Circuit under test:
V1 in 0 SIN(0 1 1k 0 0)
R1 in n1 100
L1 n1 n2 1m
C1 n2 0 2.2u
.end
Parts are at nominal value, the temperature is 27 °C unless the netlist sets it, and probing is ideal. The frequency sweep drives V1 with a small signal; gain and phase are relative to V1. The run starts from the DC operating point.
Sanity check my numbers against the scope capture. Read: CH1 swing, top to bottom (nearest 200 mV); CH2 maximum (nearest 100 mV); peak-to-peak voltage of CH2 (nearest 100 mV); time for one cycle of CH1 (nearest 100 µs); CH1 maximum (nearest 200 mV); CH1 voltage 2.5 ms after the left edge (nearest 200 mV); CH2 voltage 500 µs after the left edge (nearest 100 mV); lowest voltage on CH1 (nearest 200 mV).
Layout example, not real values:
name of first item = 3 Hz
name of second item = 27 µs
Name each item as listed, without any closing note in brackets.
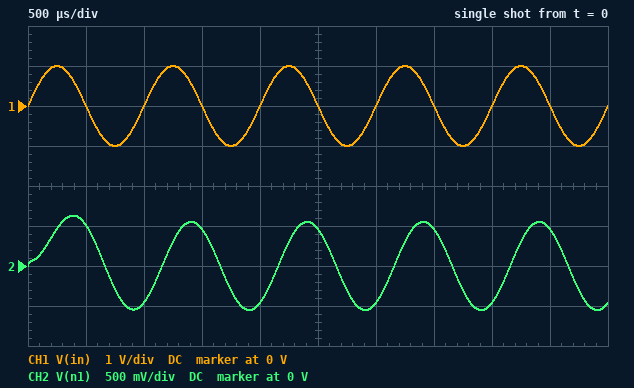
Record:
CH1 swing, top to bottom = 2.0 V
CH2 maximum = 600 mV
peak-to-peak voltage of CH2 = 1.2 V
time for one cycle of CH1 = 1.0 ms
CH1 maximum = 1.0 V
CH1 voltage 2.5 ms after the left edge = 0 V
CH2 voltage 500 µs after the left edge = 500 mV
lowest voltage on CH1 = -1.0 V
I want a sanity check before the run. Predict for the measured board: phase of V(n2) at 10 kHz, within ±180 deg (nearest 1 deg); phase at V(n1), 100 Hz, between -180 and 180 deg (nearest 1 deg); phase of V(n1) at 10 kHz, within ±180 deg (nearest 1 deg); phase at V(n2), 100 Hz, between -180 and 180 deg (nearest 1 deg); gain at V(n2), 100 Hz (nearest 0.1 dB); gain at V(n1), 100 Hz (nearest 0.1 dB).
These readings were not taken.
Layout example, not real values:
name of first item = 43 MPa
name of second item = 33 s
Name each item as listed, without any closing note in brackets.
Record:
phase of V(n2) at 10 kHz, within ±180 deg = -119 deg
phase at V(n1), 100 Hz, between -180 and 180 deg = -8 deg
phase of V(n1) at 10 kHz, within ±180 deg = 61 deg
phase at V(n2), 100 Hz, between -180 and 180 deg = -8 deg
gain at V(n2), 100 Hz = -0.1 dB
gain at V(n1), 100 Hz = -0.1 dB
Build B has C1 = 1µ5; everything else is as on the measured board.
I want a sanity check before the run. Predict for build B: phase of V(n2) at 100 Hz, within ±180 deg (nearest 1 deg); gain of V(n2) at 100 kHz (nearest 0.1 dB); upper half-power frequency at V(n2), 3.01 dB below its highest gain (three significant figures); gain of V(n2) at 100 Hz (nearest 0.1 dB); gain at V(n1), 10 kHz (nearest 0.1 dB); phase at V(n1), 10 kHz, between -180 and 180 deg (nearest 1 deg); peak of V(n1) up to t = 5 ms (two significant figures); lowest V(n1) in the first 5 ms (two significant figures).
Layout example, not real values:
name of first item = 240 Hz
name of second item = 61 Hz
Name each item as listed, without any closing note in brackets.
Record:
phase of V(n2) at 100 Hz, within ±180 deg = -5 deg
gain of V(n2) at 100 kHz = -55.5 dB
upper half-power frequency at V(n2), 3.01 dB below its highest gain = 1.14 kHz
gain of V(n2) at 100 Hz = 0 dB
gain at V(n1), 10 kHz = -6.7 dB
phase at V(n1), 10 kHz, between -180 and 180 deg = 62 deg
peak of V(n1) up to t = 5 ms = 750 mV
lowest V(n1) in the first 5 ms = -710 mV
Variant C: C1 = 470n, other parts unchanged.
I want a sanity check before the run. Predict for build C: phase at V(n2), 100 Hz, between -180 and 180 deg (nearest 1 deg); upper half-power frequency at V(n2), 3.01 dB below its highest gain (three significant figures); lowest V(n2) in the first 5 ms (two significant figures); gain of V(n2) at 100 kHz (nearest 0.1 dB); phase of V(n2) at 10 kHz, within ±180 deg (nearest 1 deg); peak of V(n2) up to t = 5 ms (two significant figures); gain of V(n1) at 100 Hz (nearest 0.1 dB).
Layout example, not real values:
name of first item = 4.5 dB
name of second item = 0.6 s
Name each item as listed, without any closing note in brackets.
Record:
phase at V(n2), 100 Hz, between -180 and 180 deg = -2 deg
upper half-power frequency at V(n2), 3.01 dB below its highest gain = 4.22 kHz
lowest V(n2) in the first 5 ms = -980 mV
gain of V(n2) at 100 kHz = -45.4 dB
phase of V(n2) at 10 kHz, within ±180 deg = -106 deg
peak of V(n2) up to t = 5 ms = 980 mV
gain of V(n1) at 100 Hz = 0 dB
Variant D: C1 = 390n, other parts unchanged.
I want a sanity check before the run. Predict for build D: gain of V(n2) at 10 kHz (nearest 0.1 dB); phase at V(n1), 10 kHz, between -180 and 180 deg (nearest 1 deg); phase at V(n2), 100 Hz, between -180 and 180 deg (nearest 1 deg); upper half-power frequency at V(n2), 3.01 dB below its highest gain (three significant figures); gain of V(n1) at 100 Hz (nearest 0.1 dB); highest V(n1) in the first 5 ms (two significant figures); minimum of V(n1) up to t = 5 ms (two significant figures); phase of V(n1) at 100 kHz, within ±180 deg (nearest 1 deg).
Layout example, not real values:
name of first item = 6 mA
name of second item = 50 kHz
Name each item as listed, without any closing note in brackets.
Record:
gain of V(n2) at 10 kHz = -8.0 dB
phase at V(n1), 10 kHz, between -180 and 180 deg = 78 deg
phase at V(n2), 100 Hz, between -180 and 180 deg = -1 deg
upper half-power frequency at V(n2), 3.01 dB below its highest gain = 5.28 kHz
gain of V(n1) at 100 Hz = 0 dB
highest V(n1) in the first 5 ms = 970 mV
minimum of V(n1) up to t = 5 ms = -970 mV
phase of V(n1) at 100 kHz, within ±180 deg = 9 deg
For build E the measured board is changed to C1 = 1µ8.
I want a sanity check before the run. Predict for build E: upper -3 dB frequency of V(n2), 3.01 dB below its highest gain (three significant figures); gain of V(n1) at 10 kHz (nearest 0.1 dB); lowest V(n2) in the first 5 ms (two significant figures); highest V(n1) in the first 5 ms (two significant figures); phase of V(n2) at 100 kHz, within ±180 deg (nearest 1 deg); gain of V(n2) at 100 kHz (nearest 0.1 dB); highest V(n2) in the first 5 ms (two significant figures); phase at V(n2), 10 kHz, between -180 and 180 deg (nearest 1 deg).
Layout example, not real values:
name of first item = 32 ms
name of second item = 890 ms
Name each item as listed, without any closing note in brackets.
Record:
upper -3 dB frequency of V(n2), 3.01 dB below its highest gain = 936 Hz
gain of V(n1) at 10 kHz = -6.5 dB
lowest V(n2) in the first 5 ms = -680 mV
highest V(n1) in the first 5 ms = 690 mV
phase of V(n2) at 100 kHz, within ±180 deg = -171 deg
gain of V(n2) at 100 kHz = -57.1 dB
highest V(n2) in the first 5 ms = 740 mV
phase at V(n2), 10 kHz, between -180 and 180 deg = -118 deg
